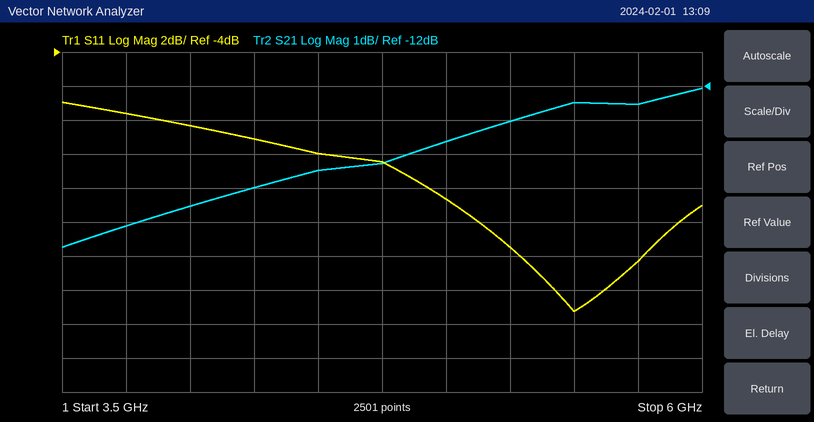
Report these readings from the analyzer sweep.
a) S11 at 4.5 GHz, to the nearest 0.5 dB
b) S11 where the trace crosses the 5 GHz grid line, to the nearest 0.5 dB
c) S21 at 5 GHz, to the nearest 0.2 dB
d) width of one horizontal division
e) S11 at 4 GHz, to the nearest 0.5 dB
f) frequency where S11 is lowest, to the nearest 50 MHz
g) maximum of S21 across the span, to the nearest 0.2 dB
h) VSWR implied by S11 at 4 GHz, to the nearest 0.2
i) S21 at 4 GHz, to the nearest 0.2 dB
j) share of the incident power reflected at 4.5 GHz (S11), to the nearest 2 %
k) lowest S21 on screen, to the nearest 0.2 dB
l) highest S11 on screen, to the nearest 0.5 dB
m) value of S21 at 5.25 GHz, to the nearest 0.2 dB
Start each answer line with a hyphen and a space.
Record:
- -10.0 dB
- -12.5 dB
- -13.6 dB
- 250 MHz
- -8.5 dB
- 5.50 GHz
- -12.0 dB
- 2.2
- -15.6 dB
- 10 %
- -16.8 dB
- -7.0 dB
- -13.0 dB
